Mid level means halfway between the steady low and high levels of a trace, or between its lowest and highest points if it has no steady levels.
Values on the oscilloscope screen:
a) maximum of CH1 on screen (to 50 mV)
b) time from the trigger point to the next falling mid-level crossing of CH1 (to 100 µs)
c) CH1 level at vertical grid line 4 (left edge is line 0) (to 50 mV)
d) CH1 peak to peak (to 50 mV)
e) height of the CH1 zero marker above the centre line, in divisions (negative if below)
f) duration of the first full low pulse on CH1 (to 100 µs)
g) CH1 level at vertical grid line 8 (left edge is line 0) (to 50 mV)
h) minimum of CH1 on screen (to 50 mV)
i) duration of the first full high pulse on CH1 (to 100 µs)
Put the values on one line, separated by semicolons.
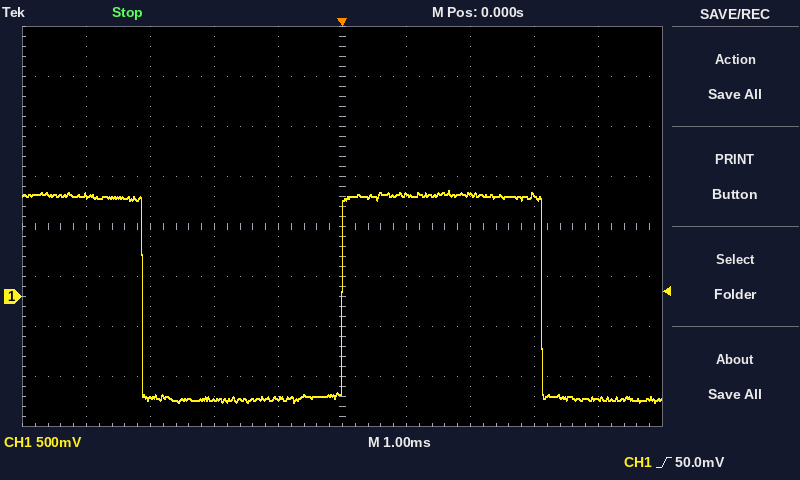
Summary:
1.05 V; 3.1 ms; -1.00 V; 2.10 V; -1.4 div; 3.1 ms; 1.00 V; -1.05 V; 3.1 ms
